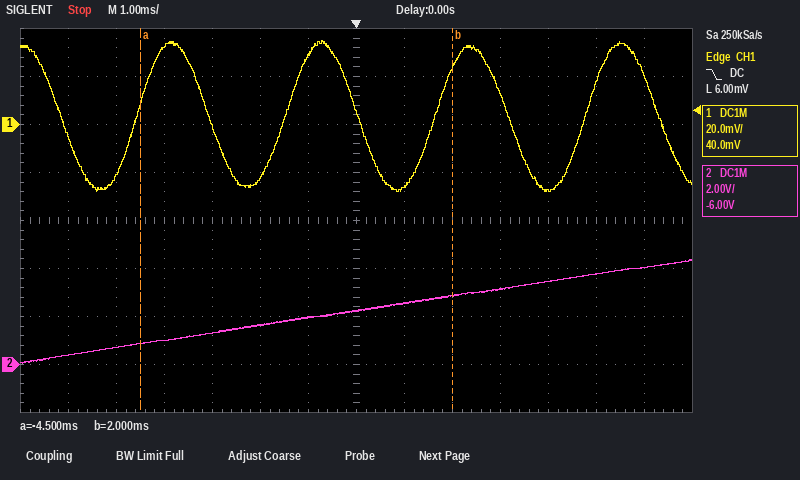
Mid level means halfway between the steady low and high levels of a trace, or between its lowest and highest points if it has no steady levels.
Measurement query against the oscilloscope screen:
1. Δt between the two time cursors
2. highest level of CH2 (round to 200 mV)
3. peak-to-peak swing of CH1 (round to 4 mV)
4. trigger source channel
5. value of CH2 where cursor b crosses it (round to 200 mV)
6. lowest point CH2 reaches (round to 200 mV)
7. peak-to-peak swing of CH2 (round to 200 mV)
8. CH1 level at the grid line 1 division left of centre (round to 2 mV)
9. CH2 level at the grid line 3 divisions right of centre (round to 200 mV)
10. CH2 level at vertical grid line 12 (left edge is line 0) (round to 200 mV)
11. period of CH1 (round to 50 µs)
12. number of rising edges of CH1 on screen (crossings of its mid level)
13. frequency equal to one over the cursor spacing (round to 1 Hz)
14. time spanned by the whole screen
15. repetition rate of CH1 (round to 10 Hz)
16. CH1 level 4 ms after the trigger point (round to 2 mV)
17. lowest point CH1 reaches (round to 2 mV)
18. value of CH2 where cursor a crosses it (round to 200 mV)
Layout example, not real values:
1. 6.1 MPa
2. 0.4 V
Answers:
1. 6.5 ms
2. 4.4 V
3. 64 mV
4. CH1
5. 2.8 V
6. 0.0 V
7. 4.4 V
8. 28 mV
9. 3.2 V
10. 3.8 V
11. 3.10 ms
12. 4
13. 154 Hz
14. 14 ms
15. 320 Hz
16. -28 mV
17. -28 mV
18. 800 mV
